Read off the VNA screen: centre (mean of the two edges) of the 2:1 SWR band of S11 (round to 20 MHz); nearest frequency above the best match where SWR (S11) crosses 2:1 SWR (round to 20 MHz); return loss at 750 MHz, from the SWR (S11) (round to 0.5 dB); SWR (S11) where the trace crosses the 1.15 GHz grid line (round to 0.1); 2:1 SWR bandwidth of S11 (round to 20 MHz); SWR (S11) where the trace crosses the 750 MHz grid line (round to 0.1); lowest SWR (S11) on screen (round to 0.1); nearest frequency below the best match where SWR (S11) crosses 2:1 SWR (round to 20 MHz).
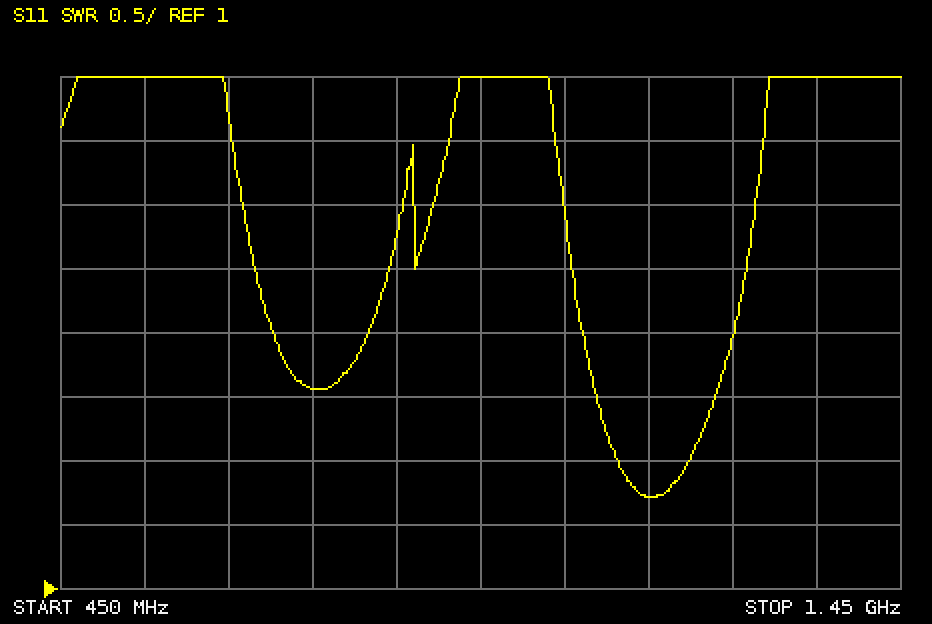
1.16 GHz
1.20 GHz
7.0 dB
1.7
80 MHz
2.6
1.7
1.12 GHz
